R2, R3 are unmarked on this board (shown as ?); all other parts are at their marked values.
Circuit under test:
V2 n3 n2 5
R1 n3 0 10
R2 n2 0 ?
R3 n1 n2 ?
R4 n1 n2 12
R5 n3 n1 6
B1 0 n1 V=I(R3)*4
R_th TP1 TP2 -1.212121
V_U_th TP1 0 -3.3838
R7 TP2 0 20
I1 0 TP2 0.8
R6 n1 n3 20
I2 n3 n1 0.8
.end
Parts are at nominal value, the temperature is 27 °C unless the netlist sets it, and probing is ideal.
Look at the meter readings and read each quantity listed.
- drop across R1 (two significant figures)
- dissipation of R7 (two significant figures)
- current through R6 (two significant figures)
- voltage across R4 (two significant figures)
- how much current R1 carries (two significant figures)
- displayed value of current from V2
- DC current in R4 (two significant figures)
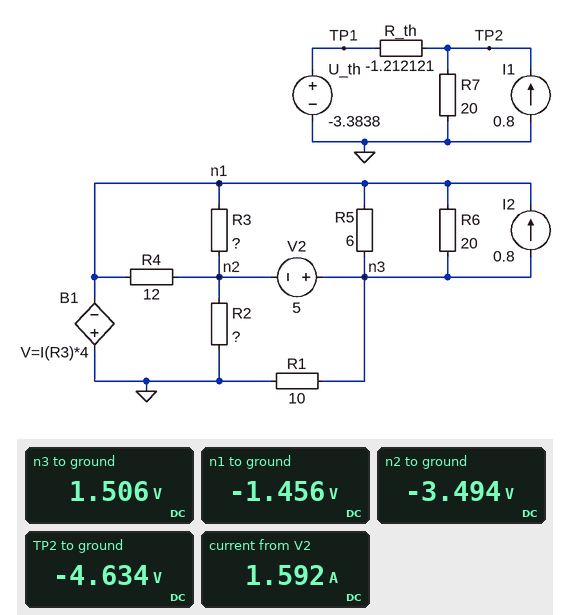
1.5 V
1.1 W
150 mA
2.0 V
150 mA
1.592 A
170 mA
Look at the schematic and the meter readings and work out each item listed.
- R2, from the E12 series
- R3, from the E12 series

3.3 Ω
5.6 Ω
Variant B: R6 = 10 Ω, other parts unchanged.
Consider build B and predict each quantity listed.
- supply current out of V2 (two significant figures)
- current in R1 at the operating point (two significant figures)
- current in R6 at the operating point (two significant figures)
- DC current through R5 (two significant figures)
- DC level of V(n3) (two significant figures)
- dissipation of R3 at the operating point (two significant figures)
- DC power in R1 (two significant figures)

1.7 A
130 mA
280 mA
470 mA
1.3 V
830 mW
170 mW
